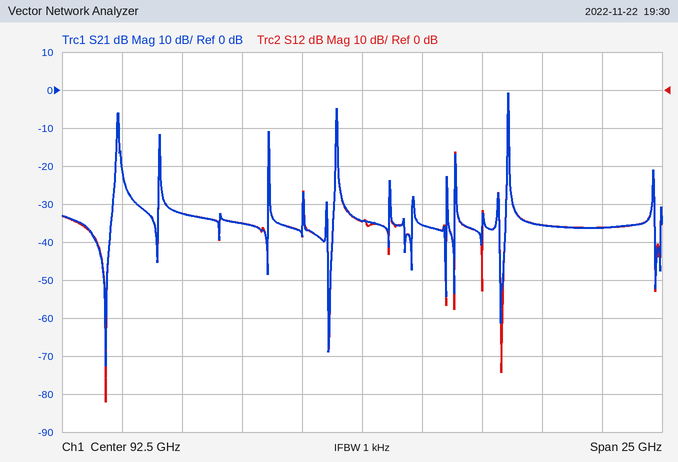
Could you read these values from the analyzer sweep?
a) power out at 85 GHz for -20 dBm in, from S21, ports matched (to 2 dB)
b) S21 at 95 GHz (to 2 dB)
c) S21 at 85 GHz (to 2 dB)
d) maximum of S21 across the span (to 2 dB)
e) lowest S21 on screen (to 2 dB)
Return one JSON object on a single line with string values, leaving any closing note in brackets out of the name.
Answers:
{"power out at 85 GHz for -20 dBm in, from S21, ports matched": "-52 dBm", "S21 at 95 GHz": "-36 dB", "S21 at 85 GHz": "-32 dB", "maximum of S21 across the span": "0 dB", "lowest S21 on screen": "-72 dB"}
